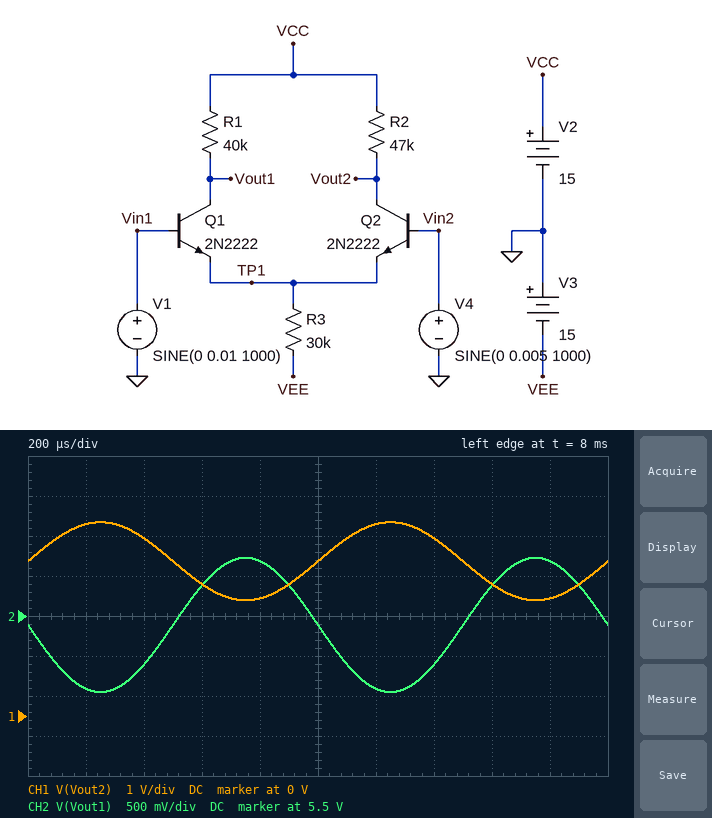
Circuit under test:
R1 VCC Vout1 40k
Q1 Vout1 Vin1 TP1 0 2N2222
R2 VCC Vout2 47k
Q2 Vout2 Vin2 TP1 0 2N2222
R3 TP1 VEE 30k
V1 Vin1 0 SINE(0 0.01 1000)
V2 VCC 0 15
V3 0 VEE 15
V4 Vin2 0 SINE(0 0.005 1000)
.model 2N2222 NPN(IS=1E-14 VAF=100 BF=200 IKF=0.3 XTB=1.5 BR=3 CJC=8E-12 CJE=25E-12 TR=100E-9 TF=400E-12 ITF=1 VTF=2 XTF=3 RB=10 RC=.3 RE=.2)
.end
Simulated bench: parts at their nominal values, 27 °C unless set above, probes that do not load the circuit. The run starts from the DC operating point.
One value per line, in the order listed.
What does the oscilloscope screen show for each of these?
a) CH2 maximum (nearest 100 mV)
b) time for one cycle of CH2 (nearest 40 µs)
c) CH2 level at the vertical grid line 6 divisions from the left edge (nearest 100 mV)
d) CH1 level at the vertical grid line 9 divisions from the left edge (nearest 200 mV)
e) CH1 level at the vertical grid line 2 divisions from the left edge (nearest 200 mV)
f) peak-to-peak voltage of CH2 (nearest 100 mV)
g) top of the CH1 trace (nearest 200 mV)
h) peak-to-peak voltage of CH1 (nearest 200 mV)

6.2 V
1.00 ms
4.6 V
3.0 V
4.4 V
1.7 V
4.8 V
2.0 V
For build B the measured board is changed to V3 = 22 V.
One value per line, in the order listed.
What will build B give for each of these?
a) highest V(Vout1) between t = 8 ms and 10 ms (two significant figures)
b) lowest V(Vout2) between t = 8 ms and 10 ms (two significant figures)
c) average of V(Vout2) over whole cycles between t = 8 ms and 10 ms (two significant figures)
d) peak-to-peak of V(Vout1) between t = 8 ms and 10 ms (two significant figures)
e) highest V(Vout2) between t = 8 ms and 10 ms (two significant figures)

830 mV
-590 mV
-480 mV
1.3 V
-120 mV
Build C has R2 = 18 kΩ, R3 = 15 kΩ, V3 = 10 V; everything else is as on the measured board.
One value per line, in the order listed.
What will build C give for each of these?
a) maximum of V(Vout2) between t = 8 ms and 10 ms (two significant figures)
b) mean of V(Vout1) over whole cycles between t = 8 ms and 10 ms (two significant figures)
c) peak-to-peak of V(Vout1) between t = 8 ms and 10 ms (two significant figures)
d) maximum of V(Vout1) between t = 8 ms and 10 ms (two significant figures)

9.7 V
2.9 V
2.2 V
4.0 V
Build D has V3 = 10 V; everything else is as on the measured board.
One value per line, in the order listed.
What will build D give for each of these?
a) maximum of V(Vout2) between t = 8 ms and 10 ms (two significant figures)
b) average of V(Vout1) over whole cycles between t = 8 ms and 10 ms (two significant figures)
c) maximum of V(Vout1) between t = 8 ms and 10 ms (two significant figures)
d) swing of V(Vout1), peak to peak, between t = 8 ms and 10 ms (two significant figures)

8.4 V
8.7 V
9.3 V
1.1 V
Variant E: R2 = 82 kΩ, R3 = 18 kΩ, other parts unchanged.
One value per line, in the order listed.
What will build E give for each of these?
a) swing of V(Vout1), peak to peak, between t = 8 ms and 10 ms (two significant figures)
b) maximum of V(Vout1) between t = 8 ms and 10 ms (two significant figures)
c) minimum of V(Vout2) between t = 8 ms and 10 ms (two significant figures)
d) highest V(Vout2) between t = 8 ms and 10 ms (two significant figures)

9.1 mV
-610 mV
-640 mV
-620 mV
